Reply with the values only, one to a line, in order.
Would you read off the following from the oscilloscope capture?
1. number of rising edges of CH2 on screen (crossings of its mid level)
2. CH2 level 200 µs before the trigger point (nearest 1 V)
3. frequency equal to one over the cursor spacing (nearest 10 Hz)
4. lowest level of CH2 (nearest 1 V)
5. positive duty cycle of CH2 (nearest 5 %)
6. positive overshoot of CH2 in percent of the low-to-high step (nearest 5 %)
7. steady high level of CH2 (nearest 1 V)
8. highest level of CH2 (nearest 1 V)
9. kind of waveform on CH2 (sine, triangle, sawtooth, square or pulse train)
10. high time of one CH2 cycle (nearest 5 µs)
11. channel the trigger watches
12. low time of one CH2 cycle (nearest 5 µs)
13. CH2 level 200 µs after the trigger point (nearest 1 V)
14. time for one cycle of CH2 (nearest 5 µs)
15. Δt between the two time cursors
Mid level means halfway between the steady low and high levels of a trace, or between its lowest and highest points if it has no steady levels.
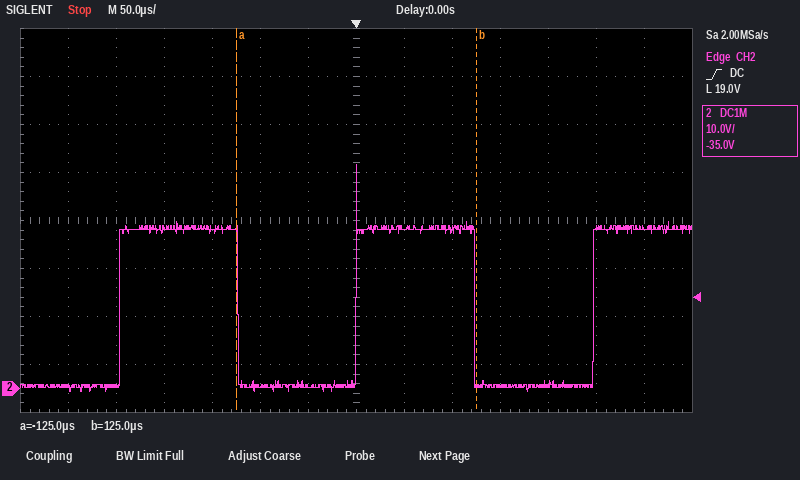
3
33 V
4.00 kHz
-1 V
50 %
40 %
33 V
47 V
square
125 µs
CH2
125 µs
1 V
245 µs
250 µs
